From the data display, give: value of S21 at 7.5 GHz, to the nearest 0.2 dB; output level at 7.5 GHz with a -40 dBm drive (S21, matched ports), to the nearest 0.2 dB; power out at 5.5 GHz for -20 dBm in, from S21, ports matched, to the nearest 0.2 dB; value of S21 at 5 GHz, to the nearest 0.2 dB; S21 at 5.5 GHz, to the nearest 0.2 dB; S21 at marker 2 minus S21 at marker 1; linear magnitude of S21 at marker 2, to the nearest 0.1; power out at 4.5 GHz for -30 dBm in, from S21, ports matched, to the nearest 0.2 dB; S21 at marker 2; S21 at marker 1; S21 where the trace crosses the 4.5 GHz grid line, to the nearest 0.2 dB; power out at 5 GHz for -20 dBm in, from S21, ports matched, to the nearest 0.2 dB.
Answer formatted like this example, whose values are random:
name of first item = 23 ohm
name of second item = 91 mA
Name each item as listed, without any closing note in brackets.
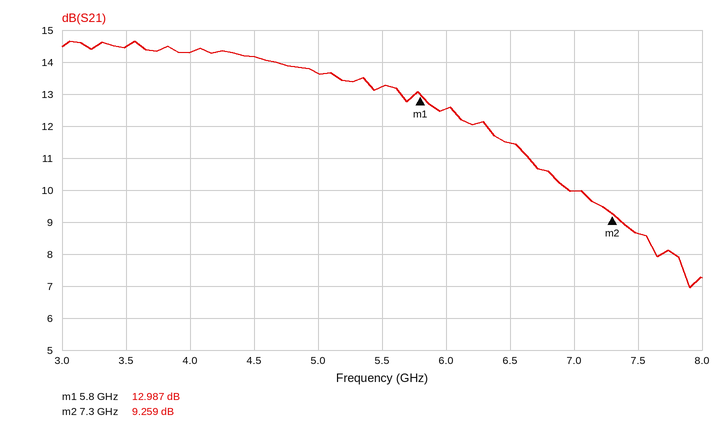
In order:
value of S21 at 7.5 GHz, to the nearest 0.2 dB = 8.6 dB
output level at 7.5 GHz with a -40 dBm drive (S21, matched ports), to the nearest 0.2 dB = -31.4 dBm
power out at 5.5 GHz for -20 dBm in, from S21, ports matched, to the nearest 0.2 dB = -6.8 dBm
value of S21 at 5 GHz, to the nearest 0.2 dB = 13.6 dB
S21 at 5.5 GHz, to the nearest 0.2 dB = 13.2 dB
S21 at marker 2 minus S21 at marker 1 = -3.728 dB
linear magnitude of S21 at marker 2, to the nearest 0.1 = 2.9
power out at 4.5 GHz for -30 dBm in, from S21, ports matched, to the nearest 0.2 dB = -15.8 dBm
S21 at marker 2 = 9.259 dB
S21 at marker 1 = 12.987 dB
S21 where the trace crosses the 4.5 GHz grid line, to the nearest 0.2 dB = 14.2 dB
power out at 5 GHz for -20 dBm in, from S21, ports matched, to the nearest 0.2 dB = -6.4 dBm
